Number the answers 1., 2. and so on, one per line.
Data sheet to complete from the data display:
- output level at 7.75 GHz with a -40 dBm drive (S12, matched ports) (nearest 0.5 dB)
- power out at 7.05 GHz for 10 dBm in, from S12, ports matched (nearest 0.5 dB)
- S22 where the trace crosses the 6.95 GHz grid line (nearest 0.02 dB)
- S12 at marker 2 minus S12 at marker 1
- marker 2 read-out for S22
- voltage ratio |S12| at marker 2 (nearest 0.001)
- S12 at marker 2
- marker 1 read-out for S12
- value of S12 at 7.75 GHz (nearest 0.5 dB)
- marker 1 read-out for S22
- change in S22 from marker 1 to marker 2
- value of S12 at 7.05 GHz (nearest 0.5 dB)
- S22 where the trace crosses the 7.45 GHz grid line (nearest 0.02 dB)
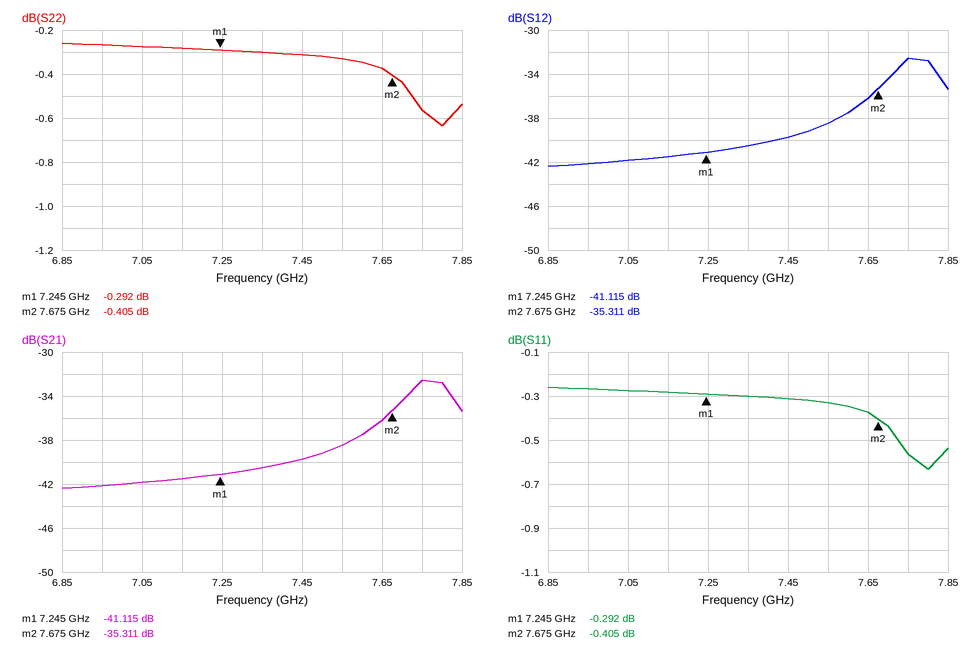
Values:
1. -72.5 dBm
2. -32.0 dBm
3. -0.26 dB
4. 5.804 dB
5. -0.405 dB
6. 0.017
7. -35.311 dB
8. -41.115 dB
9. -32.5 dB
10. -0.292 dB
11. -0.113 dB
12. -42.0 dB
13. -0.32 dB
